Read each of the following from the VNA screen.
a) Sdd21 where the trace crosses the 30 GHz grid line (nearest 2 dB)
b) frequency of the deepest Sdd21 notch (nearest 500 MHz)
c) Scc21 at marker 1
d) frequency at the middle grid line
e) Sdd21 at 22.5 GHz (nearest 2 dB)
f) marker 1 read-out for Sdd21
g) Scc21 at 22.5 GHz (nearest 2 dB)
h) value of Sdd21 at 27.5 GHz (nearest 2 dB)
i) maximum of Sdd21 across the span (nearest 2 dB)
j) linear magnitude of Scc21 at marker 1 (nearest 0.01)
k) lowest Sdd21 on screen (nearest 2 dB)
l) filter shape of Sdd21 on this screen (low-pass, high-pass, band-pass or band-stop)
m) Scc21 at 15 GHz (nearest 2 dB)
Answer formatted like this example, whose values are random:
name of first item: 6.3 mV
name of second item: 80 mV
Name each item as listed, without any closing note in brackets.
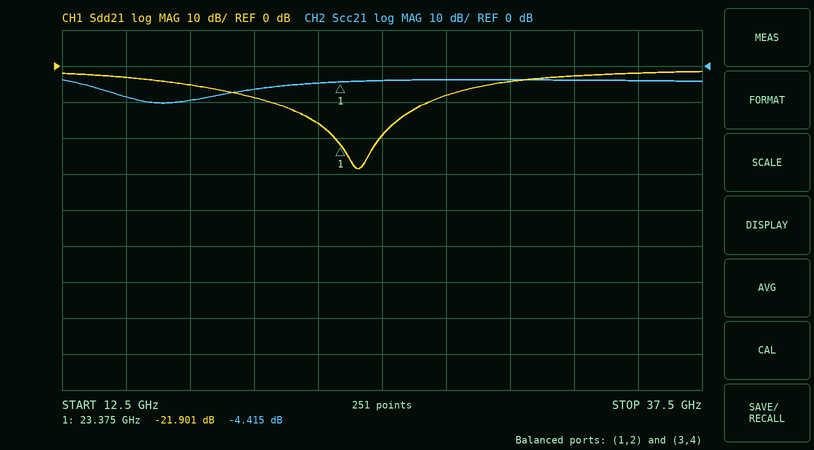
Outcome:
Sdd21 where the trace crosses the 30 GHz grid line: -4 dB
frequency of the deepest Sdd21 notch: 24.0 GHz
Scc21 at marker 1: -4.415 dB
frequency at the middle grid line: 25 GHz
Sdd21 at 22.5 GHz: -16 dB
marker 1 read-out for Sdd21: -21.901 dB
Scc21 at 22.5 GHz: -4 dB
value of Sdd21 at 27.5 GHz: -8 dB
maximum of Sdd21 across the span: -2 dB
linear magnitude of Scc21 at marker 1: 0.60
lowest Sdd21 on screen: -28 dB
filter shape of Sdd21 on this screen: band-stop
Scc21 at 15 GHz: -8 dB
